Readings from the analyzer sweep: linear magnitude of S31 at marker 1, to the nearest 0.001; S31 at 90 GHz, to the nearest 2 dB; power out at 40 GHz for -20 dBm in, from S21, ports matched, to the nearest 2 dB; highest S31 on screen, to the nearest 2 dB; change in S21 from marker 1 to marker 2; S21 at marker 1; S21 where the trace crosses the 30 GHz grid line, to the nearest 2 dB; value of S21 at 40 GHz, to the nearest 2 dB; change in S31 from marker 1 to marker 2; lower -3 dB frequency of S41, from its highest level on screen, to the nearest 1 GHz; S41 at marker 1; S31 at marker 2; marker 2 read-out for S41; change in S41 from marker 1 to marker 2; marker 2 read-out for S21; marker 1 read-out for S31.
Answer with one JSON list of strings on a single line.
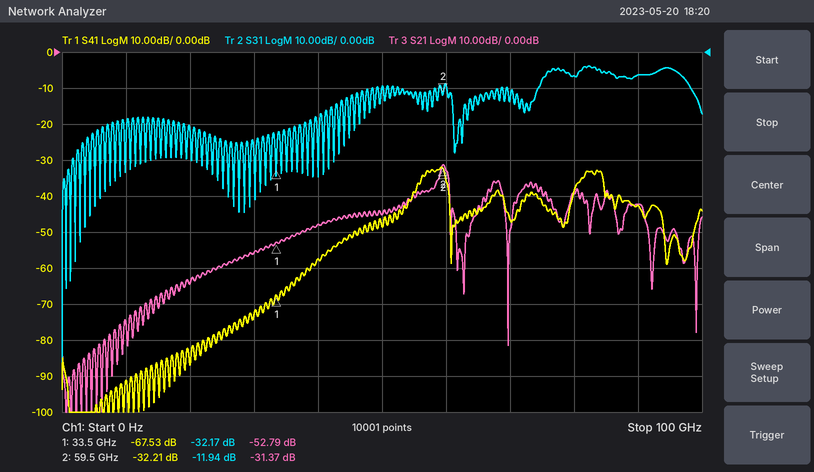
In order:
["0.025", "-6 dB", "-68 dBm", "-4 dB", "21.42 dB", "-52.79 dB", "-56 dB", "-48 dB", "20.23 dB", "56 GHz", "-67.53 dB", "-11.94 dB", "-32.21 dB", "35.32 dB", "-31.37 dB", "-32.17 dB"]
